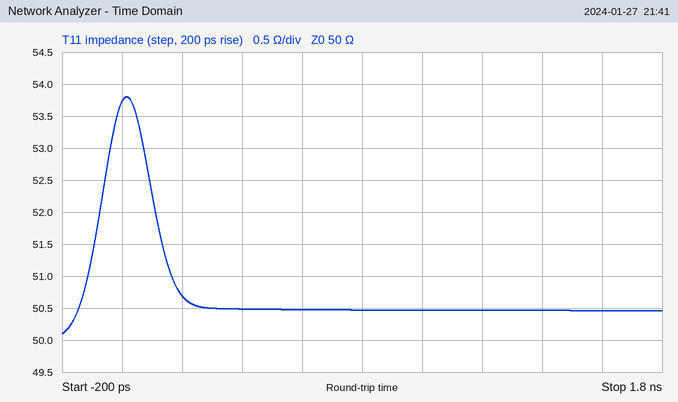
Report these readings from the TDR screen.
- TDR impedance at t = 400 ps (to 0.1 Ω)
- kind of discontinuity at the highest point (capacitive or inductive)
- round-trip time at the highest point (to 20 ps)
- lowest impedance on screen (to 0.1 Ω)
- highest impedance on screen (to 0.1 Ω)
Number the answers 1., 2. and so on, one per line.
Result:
1. 50.5 Ω
2. inductive
3. 20 ps
4. 50.1 Ω
5. 53.8 Ω
